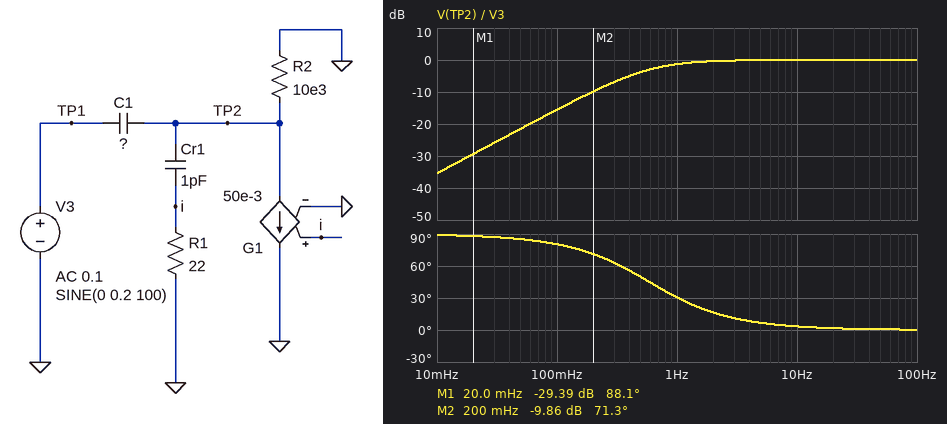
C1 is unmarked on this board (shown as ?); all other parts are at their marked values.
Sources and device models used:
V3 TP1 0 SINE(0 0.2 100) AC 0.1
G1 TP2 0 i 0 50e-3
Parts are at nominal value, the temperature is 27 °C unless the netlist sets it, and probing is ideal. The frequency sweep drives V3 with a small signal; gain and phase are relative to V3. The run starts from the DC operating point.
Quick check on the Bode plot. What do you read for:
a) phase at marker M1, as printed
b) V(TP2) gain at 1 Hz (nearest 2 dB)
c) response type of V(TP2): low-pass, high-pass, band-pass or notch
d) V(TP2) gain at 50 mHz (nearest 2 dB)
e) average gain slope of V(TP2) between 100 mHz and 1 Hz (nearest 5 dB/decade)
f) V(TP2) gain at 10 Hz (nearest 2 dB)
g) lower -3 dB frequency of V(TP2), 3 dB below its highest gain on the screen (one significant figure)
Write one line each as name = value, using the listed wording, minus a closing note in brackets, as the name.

phase at marker M1, as printed = 88.1 deg
V(TP2) gain at 1 Hz = -2 dB
response type of V(TP2): low-pass, high-pass, band-pass or notch = high-pass
V(TP2) gain at 50 mHz = -22 dB
average gain slope of V(TP2) between 100 mHz and 1 Hz = 15 dB/decade
V(TP2) gain at 10 Hz = 0 dB
lower -3 dB frequency of V(TP2), 3 dB below its highest gain on the screen = 600 mHz
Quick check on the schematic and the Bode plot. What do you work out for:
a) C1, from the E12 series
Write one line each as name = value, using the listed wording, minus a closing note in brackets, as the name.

C1, from the E12 series = 27 µF
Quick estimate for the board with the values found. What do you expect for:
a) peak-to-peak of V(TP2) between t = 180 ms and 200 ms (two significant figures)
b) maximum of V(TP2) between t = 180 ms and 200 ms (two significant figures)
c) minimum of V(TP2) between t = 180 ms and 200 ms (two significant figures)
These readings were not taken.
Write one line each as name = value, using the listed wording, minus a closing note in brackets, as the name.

peak-to-peak of V(TP2) between t = 180 ms and 200 ms = 400 mV
maximum of V(TP2) between t = 180 ms and 200 ms = 200 mV
minimum of V(TP2) between t = 180 ms and 200 ms = -200 mV
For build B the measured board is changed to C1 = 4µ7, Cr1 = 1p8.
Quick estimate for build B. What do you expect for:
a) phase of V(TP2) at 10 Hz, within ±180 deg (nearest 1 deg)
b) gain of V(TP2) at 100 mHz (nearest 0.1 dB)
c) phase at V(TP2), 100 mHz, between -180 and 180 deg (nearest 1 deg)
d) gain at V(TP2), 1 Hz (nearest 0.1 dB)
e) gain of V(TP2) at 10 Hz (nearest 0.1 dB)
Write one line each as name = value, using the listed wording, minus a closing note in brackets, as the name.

phase of V(TP2) at 10 Hz, within ±180 deg = 19 deg
gain of V(TP2) at 100 mHz = -30.6 dB
phase at V(TP2), 100 mHz, between -180 and 180 deg = 88 deg
gain at V(TP2), 1 Hz = -11.0 dB
gain of V(TP2) at 10 Hz = -0.5 dB
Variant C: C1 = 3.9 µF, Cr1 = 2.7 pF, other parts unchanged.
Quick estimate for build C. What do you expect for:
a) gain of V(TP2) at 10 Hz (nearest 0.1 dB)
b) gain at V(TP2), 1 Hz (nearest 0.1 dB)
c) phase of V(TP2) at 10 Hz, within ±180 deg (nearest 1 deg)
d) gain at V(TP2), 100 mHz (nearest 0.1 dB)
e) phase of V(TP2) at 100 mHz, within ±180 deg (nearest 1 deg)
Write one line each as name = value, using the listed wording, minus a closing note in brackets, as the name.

gain of V(TP2) at 10 Hz = -0.7 dB
gain at V(TP2), 1 Hz = -12.5 dB
phase of V(TP2) at 10 Hz, within ±180 deg = 22 deg
gain at V(TP2), 100 mHz = -32.2 dB
phase of V(TP2) at 100 mHz, within ±180 deg = 89 deg
